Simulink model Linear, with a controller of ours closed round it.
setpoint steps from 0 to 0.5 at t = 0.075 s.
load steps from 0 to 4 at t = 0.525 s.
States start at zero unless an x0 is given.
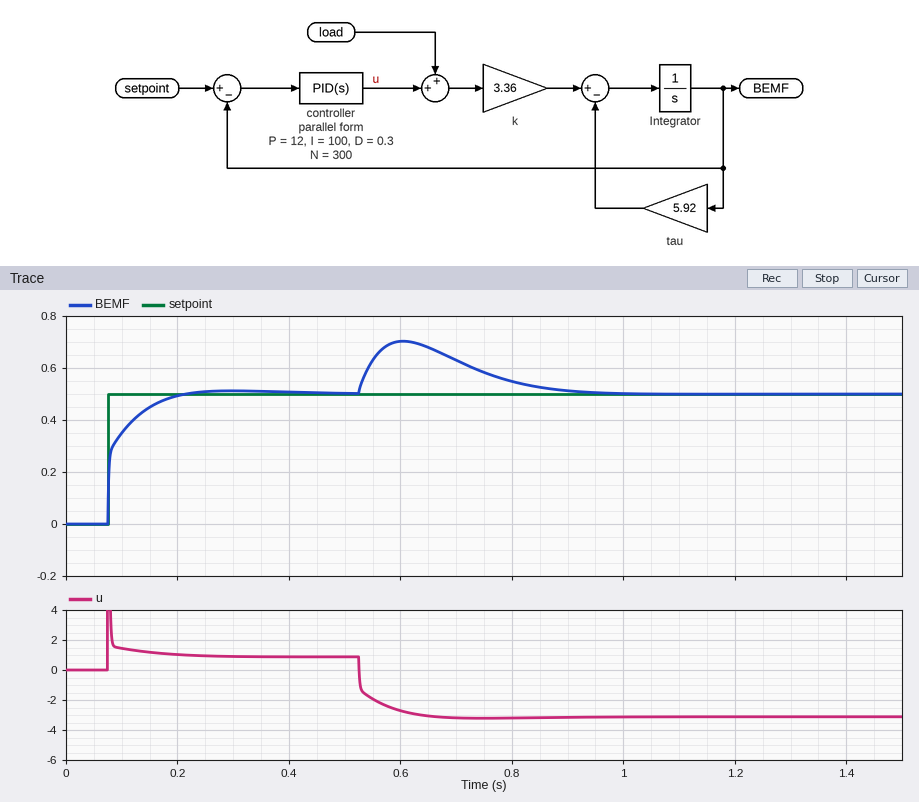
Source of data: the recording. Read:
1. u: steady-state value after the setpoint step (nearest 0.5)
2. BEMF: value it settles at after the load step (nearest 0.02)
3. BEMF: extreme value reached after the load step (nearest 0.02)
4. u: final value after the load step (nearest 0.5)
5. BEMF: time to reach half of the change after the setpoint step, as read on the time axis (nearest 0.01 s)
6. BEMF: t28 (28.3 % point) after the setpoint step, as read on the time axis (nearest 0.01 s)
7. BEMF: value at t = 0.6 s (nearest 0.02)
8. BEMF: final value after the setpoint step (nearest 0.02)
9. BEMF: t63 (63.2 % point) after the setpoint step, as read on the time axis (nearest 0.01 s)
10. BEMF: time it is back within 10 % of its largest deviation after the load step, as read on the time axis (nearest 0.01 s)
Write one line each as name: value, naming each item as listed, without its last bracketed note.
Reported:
u: steady-state value after the setpoint step: 1.0
BEMF: value it settles at after the load step: 0.50
BEMF: extreme value reached after the load step: 0.70
u: final value after the load step: -3.0
BEMF: time to reach half of the change after the setpoint step, as read on the time axis: 0.08 s
BEMF: t28 (28.3 % point) after the setpoint step, as read on the time axis: 0.08 s
BEMF: value at t = 0.6 s: 0.70
BEMF: final value after the setpoint step: 0.50
BEMF: t63 (63.2 % point) after the setpoint step, as read on the time axis: 0.09 s
BEMF: time it is back within 10 % of its largest deviation after the load step, as read on the time axis: 0.87 s
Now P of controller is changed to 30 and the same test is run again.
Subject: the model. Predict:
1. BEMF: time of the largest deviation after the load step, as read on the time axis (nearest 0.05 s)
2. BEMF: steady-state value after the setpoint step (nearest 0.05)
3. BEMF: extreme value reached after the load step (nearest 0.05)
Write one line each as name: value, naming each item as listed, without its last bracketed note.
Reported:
BEMF: time of the largest deviation after the load step, as read on the time axis: 0.60 s
BEMF: steady-state value after the setpoint step: 0.50
BEMF: extreme value reached after the load step: 0.60
